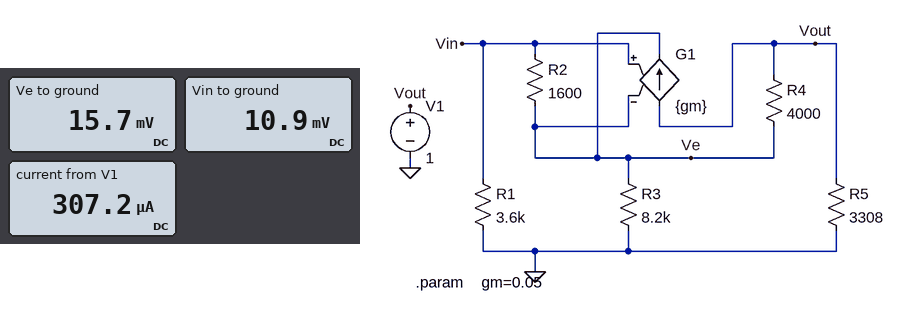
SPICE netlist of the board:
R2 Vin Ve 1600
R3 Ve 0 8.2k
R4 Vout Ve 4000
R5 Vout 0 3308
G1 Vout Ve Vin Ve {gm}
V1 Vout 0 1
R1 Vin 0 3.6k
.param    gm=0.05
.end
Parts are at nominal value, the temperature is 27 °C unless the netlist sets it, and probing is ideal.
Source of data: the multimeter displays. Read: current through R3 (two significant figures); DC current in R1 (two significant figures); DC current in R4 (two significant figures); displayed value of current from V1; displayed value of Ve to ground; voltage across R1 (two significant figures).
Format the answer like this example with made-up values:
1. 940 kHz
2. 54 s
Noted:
1. 1.9 µA
2. 3.0 µA
3. 250 µA
4. 307.2 µA
5. 15.7 mV
6. 11 mV
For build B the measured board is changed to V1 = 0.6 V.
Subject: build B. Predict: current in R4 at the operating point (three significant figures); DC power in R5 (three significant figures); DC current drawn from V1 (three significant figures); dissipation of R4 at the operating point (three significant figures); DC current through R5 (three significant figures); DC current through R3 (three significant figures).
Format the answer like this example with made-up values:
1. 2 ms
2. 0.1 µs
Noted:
1. 148 µA
2. 109 µW
3. 184 µA
4. 87.2 µW
5. 181 µA
6. 1.15 µA
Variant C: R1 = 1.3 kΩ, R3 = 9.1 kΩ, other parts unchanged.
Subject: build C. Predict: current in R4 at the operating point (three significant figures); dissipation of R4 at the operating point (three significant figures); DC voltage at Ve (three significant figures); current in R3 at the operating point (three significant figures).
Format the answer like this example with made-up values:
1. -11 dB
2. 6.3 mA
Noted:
1. 248 µA
2. 246 µW
3. 8.84 mV
4. 971 nA
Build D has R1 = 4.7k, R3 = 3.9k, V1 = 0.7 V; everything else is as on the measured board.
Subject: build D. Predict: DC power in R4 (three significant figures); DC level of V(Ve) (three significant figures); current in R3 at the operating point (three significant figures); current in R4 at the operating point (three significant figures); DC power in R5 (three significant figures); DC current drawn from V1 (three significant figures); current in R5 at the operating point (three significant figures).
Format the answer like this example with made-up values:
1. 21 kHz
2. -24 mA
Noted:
1. 118 µW
2. 13.1 mV
3. 3.36 µA
4. 172 µA
5. 148 µW
6. 217 µA
7. 212 µA
